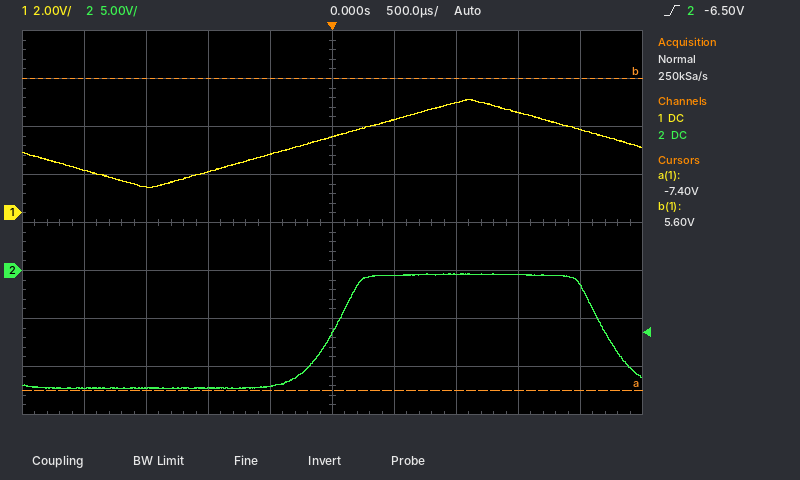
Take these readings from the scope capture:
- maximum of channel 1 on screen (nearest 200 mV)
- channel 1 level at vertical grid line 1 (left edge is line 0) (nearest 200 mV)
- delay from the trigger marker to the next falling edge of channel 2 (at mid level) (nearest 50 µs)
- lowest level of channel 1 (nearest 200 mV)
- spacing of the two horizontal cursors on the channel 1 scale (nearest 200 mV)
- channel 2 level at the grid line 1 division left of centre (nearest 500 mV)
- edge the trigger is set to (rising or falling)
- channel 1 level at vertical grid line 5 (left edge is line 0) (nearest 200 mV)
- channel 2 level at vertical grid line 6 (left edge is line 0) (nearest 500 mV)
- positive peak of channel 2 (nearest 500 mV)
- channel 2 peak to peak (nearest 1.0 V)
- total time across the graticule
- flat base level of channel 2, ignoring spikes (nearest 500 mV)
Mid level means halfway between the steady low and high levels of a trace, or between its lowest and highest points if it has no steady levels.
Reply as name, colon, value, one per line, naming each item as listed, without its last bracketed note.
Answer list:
maximum of channel 1 on screen: 4.8 V
channel 1 level at vertical grid line 1 (left edge is line 0): 1.8 V
delay from the trigger marker to the next falling edge of channel 2 (at mid level): 2.20 ms
lowest level of channel 1: 1.0 V
spacing of the two horizontal cursors on the channel 1 scale: 13.0 V
channel 2 level at the grid line 1 division left of centre: -12.0 V
edge the trigger is set to: rising
channel 1 level at vertical grid line 5 (left edge is line 0): 3.2 V
channel 2 level at vertical grid line 6 (left edge is line 0): -500 mV
positive peak of channel 2: -500 mV
channel 2 peak to peak: 12.0 V
total time across the graticule: 5 ms
flat base level of channel 2, ignoring spikes: -12.0 V
